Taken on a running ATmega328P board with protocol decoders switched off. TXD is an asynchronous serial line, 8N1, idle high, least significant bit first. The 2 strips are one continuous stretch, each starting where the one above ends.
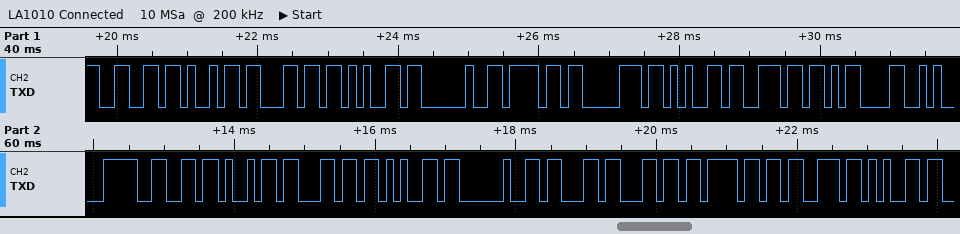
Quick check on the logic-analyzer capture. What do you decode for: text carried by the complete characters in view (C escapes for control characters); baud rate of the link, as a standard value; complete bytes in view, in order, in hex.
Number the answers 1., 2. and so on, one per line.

1. "file open\r\nfile close"
2. 9600 baud
3. 66 69 6C 65 20 6F 70 65 6E 0D 0A 66 69 6C 65 20 63 6C 6F 73 65
